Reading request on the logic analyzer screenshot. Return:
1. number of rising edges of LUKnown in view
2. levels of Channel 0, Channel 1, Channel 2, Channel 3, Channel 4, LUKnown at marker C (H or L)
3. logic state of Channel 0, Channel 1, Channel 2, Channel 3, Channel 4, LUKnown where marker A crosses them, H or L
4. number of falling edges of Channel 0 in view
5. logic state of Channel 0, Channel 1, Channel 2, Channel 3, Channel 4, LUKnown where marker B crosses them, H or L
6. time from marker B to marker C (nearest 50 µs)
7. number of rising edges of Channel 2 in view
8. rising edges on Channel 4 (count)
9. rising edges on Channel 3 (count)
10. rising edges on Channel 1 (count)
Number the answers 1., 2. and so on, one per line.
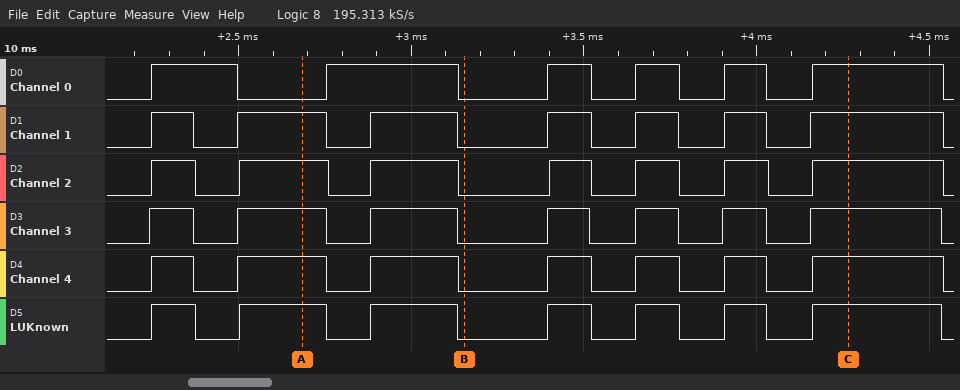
1. 7
2. Channel 0=H, Channel 1=H, Channel 2=H, Channel 3=H, Channel 4=H, LUKnown=H
3. Channel 0=L, Channel 1=H, Channel 2=H, Channel 3=H, Channel 4=H, LUKnown=H
4. 6
5. Channel 0=L, Channel 1=L, Channel 2=L, Channel 3=L, Channel 4=L, LUKnown=L
6. 1100 µs
7. 7
8. 7
9. 7
10. 7
